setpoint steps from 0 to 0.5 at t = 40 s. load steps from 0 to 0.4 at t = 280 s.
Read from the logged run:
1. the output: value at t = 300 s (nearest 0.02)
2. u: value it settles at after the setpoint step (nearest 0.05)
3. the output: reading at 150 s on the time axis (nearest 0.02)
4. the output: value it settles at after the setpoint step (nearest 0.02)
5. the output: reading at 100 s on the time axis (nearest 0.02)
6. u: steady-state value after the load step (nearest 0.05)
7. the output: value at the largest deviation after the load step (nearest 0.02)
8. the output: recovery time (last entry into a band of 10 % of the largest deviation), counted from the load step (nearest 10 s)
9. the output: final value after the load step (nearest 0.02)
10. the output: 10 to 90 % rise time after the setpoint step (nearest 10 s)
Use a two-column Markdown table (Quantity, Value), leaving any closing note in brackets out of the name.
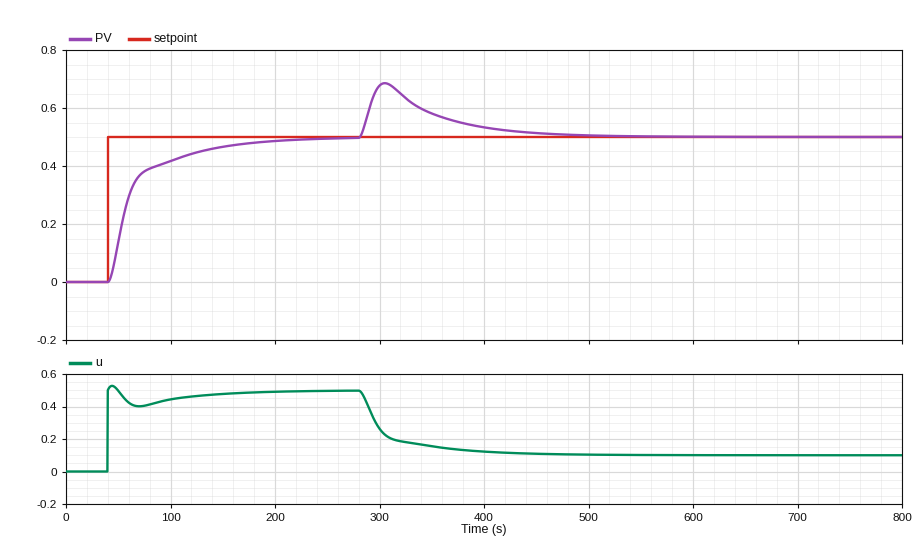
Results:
| Quantity | Value |
|---|---|
| the output: value at t = 300 s | 0.68 |
| u: value it settles at after the setpoint step | 0.50 |
| the output: reading at 150 s on the time axis | 0.46 |
| the output: value it settles at after the setpoint step | 0.50 |
| the output: reading at 100 s on the time axis | 0.42 |
| u: steady-state value after the load step | 0.10 |
| the output: value at the largest deviation after the load step | 0.68 |
| the output: recovery time (last entry into a band of 10 % of the largest deviation), counted from the load step | 150 s |
| the output: final value after the load step | 0.50 |
| the output: 10 to 90 % rise time after the setpoint step | 80 s |
